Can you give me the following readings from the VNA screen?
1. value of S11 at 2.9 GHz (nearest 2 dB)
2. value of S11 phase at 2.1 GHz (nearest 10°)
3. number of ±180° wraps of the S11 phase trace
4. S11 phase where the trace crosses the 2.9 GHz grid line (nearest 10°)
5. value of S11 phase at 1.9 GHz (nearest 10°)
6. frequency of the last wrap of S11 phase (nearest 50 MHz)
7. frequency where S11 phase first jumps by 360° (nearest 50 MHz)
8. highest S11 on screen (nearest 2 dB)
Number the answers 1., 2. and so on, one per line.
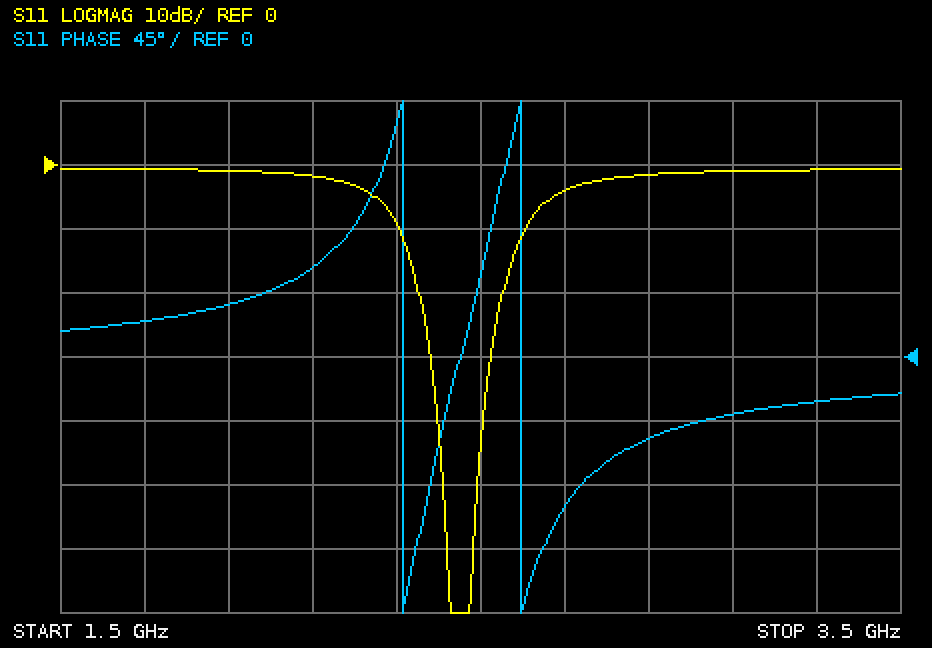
1. -2 dB
2. 60°
3. 2
4. -60°
5. 40°
6. 2.60 GHz
7. 2.30 GHz
8. 0 dB
